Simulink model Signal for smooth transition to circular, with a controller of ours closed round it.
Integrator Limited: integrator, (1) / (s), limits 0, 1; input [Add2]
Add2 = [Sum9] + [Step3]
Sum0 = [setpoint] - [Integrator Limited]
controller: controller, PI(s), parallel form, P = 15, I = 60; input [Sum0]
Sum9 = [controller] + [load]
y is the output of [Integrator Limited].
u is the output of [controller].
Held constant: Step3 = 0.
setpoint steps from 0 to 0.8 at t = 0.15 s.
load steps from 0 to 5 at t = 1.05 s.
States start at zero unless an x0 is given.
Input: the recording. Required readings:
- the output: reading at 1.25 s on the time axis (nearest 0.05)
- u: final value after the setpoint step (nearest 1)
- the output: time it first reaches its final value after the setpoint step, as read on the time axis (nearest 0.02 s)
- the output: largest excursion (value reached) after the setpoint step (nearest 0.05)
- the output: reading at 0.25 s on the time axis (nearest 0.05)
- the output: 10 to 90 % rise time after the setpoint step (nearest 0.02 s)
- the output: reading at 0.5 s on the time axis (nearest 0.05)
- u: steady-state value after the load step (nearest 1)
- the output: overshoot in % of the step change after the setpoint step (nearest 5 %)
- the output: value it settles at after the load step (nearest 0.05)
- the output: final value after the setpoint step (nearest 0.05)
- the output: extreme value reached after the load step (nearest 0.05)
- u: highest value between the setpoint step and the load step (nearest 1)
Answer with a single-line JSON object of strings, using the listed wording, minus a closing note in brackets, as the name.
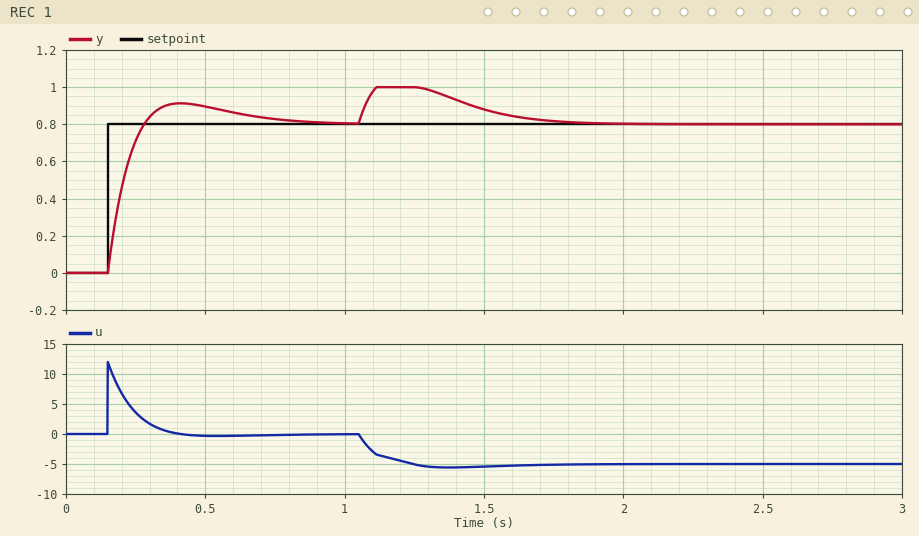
{"the output: reading at 1.25 s on the time axis": "1.00", "u: final value after the setpoint step": "0", "the output: time it first reaches its final value after the setpoint step, as read on the time axis": "0.28 s", "the output: largest excursion (value reached) after the setpoint step": "0.90", "the output: reading at 0.25 s on the time axis": "0.70", "the output: 10 to 90 % rise time after the setpoint step": "0.10 s", "the output: reading at 0.5 s on the time axis": "0.90", "u: steady-state value after the load step": "-5", "the output: overshoot in % of the step change after the setpoint step": "15 %", "the output: value it settles at after the load step": "0.80", "the output: final value after the setpoint step": "0.80", "the output: extreme value reached after the load step": "1.00", "u: highest value between the setpoint step and the load step": "12"}
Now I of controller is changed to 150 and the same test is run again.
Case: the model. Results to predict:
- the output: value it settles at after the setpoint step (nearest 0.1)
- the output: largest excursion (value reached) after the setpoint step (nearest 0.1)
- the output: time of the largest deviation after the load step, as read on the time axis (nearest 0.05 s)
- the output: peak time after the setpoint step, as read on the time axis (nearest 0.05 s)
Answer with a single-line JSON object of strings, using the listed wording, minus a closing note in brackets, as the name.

{"the output: value it settles at after the setpoint step": "0.8", "the output: largest excursion (value reached) after the setpoint step": "1.0", "the output: time of the largest deviation after the load step, as read on the time axis": "1.15 s", "the output: peak time after the setpoint step, as read on the time axis": "0.35 s"}
